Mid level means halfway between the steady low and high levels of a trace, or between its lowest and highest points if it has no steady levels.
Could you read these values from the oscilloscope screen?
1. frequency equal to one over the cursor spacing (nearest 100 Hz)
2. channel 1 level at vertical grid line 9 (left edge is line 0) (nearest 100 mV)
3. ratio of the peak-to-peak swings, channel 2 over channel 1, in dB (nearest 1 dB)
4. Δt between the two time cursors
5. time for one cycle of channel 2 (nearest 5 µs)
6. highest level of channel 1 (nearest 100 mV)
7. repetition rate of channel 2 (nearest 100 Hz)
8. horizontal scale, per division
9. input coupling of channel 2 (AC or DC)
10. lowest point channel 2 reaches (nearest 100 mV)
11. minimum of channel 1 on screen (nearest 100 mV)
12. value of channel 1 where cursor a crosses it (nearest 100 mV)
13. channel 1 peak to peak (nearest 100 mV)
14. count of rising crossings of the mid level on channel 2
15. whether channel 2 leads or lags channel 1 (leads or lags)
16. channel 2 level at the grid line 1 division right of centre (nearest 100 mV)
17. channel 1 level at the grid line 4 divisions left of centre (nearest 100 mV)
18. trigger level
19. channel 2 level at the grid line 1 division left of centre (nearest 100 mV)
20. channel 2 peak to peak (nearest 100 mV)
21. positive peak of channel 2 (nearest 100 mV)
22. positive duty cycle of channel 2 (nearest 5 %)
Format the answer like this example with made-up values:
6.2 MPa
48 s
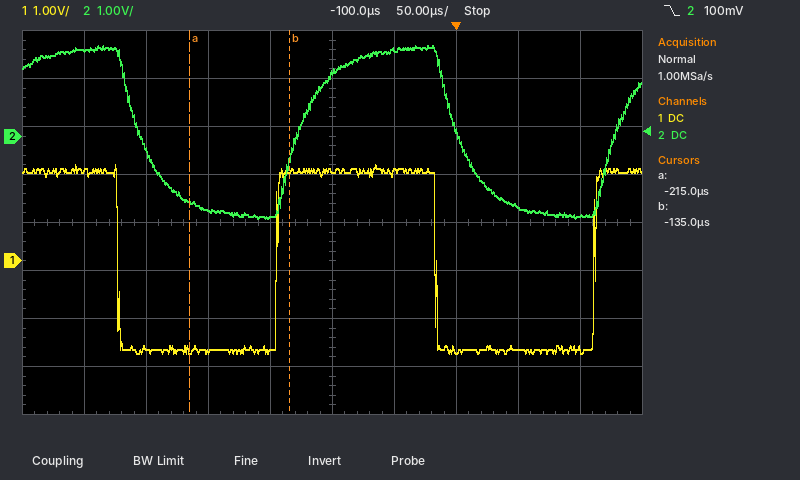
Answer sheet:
12.5 kHz
-1.8 V
-1 dB
80 µs
255 µs
2.0 V
3.9 kHz
50 µs
DC
-1.7 V
-1.9 V
-1.8 V
3.9 V
2
lags
1.8 V
1.9 V
100 mV
-1.7 V
3.6 V
1.9 V
50 %
